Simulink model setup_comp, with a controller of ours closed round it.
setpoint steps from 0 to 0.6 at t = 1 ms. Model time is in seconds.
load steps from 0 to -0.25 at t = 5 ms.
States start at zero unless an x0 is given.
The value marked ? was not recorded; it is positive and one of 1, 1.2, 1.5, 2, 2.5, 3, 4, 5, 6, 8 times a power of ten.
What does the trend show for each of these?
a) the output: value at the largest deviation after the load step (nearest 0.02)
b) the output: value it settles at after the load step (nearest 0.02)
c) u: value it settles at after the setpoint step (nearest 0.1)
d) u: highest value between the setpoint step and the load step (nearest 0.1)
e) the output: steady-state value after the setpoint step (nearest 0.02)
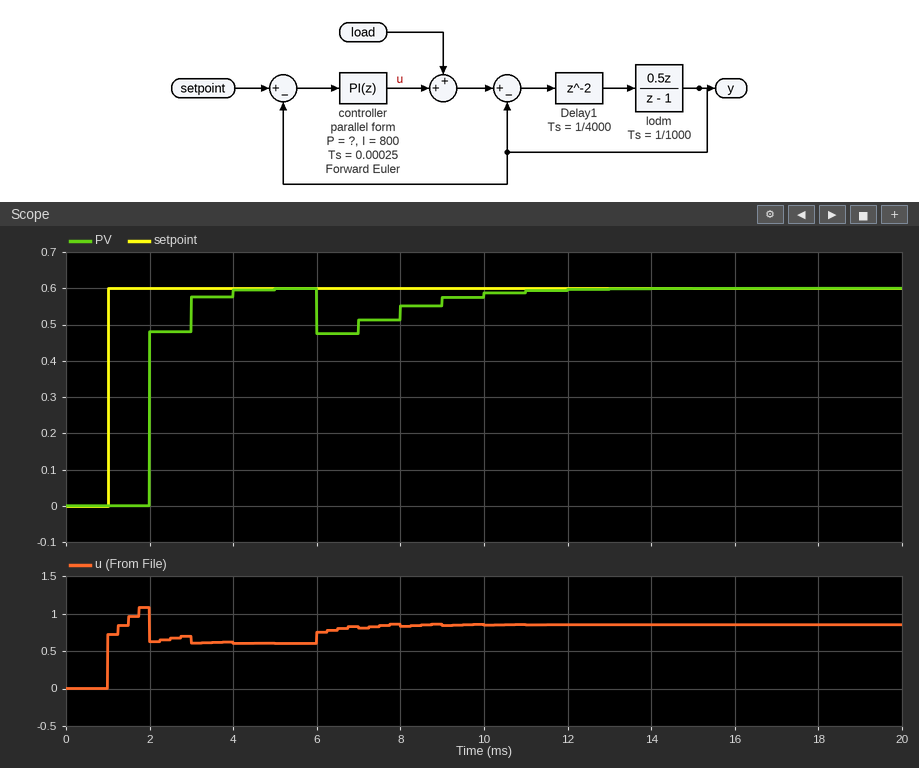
0.48
0.60
0.6
1.1
0.60
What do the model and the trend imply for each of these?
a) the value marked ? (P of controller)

1.2
